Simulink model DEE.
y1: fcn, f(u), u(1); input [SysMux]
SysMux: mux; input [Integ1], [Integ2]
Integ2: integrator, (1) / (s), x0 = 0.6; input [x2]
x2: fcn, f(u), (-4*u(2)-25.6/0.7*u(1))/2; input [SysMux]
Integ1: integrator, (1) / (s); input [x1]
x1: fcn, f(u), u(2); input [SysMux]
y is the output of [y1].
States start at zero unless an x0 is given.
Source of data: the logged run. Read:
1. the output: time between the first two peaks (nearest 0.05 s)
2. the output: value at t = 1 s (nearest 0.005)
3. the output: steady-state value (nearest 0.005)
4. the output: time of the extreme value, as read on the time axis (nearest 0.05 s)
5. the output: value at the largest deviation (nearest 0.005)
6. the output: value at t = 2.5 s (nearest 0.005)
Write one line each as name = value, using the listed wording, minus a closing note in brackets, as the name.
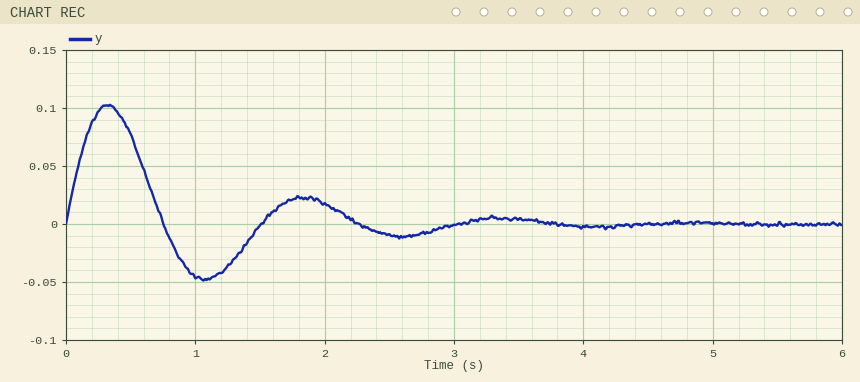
the output: time between the first two peaks = 1.50 s
the output: value at t = 1 s = -0.045
the output: steady-state value = 0.000
the output: time of the extreme value, as read on the time axis = 0.30 s
the output: value at the largest deviation = 0.100
the output: value at t = 2.5 s = -0.010
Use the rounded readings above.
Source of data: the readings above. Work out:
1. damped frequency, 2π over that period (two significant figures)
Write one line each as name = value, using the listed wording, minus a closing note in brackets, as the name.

damped frequency, 2π over that period = 4.2 rad/s
